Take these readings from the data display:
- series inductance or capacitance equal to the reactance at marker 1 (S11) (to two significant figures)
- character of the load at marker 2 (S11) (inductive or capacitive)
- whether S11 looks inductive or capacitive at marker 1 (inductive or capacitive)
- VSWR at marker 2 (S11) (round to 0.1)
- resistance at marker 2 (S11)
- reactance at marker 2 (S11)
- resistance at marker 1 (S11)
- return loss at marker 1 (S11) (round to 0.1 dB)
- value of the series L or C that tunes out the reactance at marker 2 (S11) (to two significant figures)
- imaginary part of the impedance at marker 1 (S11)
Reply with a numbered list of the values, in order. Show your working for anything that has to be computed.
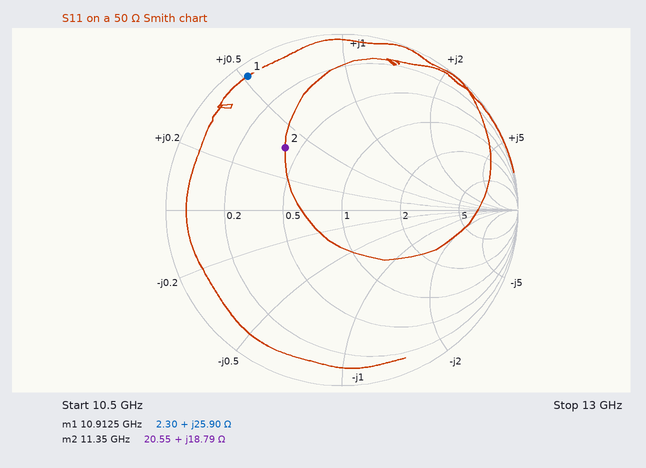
1. L = 25.9 Ω/(2π × 10.9125 GHz) ≈ 378 pH, so 380 pH to two significant figures
2. inductive
3. inductive
4. 2.8
5. 20.55 Ω
6. +18.79 Ω
7. 2.30 Ω
8. 0.6 dB
9. C = 1/(2π × 11.35 GHz × 18.79 Ω) ≈ 746 fF, so 750 fF to two significant figures
10. +25.90 Ω
